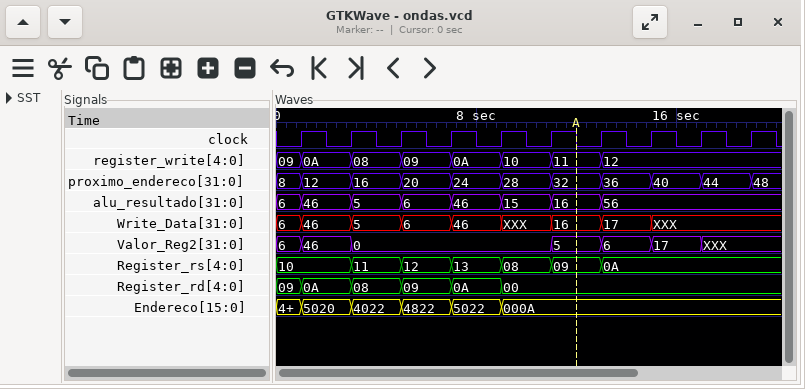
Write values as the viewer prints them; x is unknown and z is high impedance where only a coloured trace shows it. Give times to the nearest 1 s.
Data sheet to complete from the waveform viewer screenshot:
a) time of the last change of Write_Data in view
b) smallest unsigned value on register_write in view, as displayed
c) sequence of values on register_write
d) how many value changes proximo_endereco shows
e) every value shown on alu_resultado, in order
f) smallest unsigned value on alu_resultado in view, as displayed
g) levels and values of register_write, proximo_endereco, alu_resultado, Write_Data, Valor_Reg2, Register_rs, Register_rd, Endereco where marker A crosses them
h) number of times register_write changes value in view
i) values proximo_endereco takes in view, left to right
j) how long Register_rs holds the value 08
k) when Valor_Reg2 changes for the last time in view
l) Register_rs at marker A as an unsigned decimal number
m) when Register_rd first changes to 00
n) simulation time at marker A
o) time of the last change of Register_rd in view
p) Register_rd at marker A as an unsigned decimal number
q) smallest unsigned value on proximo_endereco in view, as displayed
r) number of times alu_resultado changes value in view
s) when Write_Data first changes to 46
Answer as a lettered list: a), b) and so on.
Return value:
a) 15 s
b) 08
c) 09, 0A, 08, 09, 0A, 10, 11, 12
d) 10
e) 6, 46, 5, 6, 46, 15, 16, 56
f) 5
g) register_write=11, proximo_endereco=32, alu_resultado=16, Write_Data=16, Valor_Reg2=5, Register_rs=09, Register_rd=00, Endereco=000A
h) 7
i) 8, 12, 16, 20, 24, 28, 32, 36, 40, 44, 48
j) 2 s
k) 17 s
l) 9
m) 9 s
n) 12 s
o) 9 s
p) 0
q) 8
r) 7
s) 1 s
